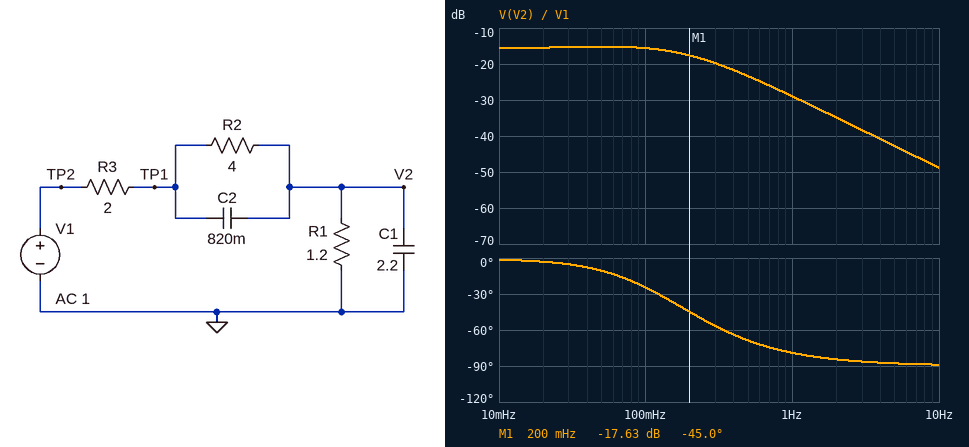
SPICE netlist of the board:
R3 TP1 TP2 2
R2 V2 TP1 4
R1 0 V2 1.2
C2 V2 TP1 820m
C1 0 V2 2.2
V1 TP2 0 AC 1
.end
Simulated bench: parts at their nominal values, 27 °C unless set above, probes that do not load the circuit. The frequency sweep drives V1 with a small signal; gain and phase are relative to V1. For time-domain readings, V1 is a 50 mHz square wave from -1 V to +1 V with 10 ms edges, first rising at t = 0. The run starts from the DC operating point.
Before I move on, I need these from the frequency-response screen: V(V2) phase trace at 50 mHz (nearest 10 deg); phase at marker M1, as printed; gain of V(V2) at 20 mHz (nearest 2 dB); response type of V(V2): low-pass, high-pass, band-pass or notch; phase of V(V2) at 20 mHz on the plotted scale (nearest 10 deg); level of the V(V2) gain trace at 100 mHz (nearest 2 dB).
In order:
-10 deg
-45.0 deg
-16 dB
low-pass
0 deg
-16 dB
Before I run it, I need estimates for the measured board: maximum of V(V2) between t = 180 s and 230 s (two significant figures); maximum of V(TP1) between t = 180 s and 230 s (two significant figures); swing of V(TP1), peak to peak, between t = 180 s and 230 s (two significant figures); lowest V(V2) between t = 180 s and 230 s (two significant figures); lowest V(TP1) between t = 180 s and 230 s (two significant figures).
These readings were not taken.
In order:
180 mV
720 mV
1.4 V
-180 mV
-720 mV
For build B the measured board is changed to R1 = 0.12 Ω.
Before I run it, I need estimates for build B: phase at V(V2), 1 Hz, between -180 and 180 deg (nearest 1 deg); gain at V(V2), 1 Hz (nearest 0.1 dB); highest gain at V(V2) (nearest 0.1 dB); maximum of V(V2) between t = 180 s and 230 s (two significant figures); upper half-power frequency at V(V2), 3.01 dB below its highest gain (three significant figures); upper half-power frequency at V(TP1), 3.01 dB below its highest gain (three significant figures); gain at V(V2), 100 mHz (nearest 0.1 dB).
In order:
-52 deg
-30.4 dB
-26.6 dB
63 mV
869 mHz
145 mHz
-28.9 dB
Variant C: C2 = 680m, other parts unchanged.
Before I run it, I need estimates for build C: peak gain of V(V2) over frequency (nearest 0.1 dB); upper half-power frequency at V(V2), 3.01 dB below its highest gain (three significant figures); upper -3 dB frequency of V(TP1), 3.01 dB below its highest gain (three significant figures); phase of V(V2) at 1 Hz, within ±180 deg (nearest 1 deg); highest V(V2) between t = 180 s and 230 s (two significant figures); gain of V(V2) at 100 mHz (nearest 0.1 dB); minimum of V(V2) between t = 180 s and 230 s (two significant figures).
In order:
-15.6 dB
221 mHz
212 mHz
-78 deg
170 mV
-16.3 dB
-170 mV
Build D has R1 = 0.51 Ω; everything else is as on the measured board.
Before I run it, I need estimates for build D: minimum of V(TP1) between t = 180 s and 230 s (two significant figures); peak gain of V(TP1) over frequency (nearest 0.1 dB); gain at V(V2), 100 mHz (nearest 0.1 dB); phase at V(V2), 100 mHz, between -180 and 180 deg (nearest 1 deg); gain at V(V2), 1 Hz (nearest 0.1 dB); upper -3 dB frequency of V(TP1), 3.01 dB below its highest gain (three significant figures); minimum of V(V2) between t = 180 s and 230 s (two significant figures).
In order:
-690 mV
-3.2 dB
-18.7 dB
-5 deg
-29.1 dB
175 mHz
-140 mV
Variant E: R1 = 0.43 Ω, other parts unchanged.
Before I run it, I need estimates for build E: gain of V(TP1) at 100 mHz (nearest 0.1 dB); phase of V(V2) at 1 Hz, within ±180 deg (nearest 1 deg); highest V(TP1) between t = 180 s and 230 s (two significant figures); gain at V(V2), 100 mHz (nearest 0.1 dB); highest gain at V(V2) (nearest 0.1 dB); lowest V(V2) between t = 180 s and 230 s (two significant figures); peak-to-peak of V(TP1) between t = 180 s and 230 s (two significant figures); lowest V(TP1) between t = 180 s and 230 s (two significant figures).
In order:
-4.7 dB
-73 deg
690 mV
-19.6 dB
-19.3 dB
-130 mV
1.4 V
-690 mV
